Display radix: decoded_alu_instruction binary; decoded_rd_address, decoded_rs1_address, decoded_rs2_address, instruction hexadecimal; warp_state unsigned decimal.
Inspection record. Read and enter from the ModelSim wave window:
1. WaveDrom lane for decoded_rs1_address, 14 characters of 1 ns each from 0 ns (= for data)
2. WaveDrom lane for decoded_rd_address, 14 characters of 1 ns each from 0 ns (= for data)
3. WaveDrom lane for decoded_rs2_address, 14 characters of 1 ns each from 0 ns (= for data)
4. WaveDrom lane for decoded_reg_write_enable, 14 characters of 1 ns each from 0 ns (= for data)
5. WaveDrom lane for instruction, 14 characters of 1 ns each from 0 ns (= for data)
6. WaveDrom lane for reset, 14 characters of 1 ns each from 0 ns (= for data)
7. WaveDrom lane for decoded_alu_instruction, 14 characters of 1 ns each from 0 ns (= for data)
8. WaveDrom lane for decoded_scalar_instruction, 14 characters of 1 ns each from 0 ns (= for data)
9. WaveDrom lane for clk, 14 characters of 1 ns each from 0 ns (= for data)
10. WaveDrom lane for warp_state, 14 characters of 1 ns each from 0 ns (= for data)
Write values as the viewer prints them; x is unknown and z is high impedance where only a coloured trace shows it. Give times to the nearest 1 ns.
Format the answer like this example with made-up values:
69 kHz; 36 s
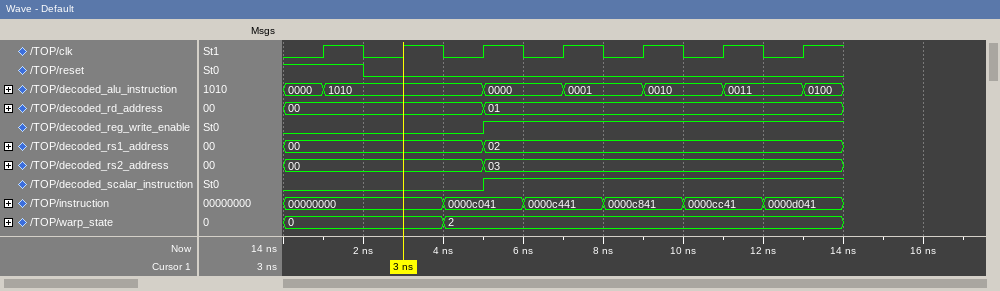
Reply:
{name: 'decoded_rs1_address', wave: '=....=........', data: '00 02'}; {name: 'decoded_rd_address', wave: '=....=........', data: '00 01'}; {name: 'decoded_rs2_address', wave: '=....=........', data: '00 03'}; {name: 'decoded_reg_write_enable', wave: '0....1........'}; {name: 'instruction', wave: '=...=.=.=.=.=.', data: '00000000 0000c041 0000c441 0000c841 0000cc41 0000d041'}; {name: 'reset', wave: '1.0...........'}; {name: 'decoded_alu_instruction', wave: '==...=.=.=.=.=', data: '0000 1010 0000 0001 0010 0011 0100'}; {name: 'decoded_scalar_instruction', wave: '0....1........'}; {name: 'clk', wave: '01010101010101'}; {name: 'warp_state', wave: '=...=.........', data: '0 2'}
